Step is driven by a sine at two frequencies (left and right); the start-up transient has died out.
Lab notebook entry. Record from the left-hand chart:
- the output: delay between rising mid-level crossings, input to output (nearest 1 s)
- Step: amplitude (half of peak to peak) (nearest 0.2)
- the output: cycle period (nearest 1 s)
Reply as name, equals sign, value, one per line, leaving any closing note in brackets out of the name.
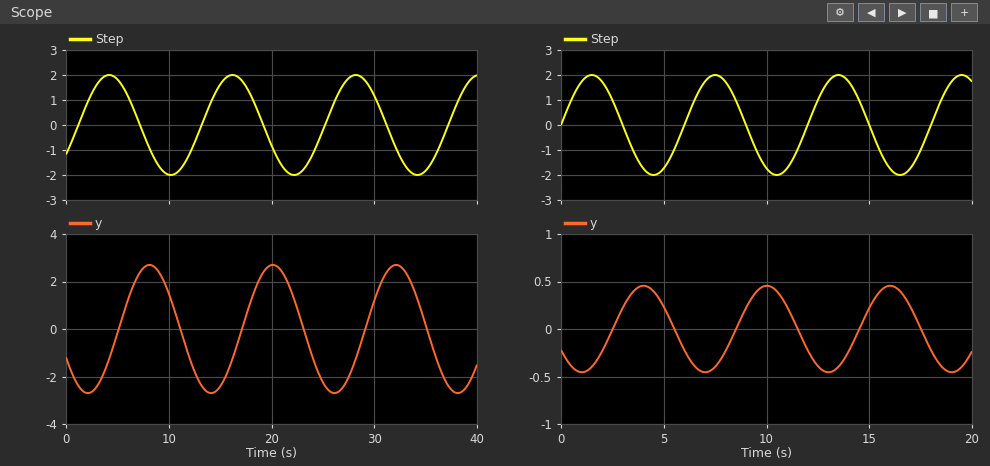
the output: delay between rising mid-level crossings, input to output = 4 s
Step: amplitude (half of peak to peak) = 2.0
the output: cycle period = 12 s
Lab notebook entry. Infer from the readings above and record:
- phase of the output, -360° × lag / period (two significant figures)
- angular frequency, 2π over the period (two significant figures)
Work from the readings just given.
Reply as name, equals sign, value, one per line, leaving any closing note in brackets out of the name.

phase of the output, -360° × lag / period = -120°
angular frequency, 2π over the period = 0.52 rad/s
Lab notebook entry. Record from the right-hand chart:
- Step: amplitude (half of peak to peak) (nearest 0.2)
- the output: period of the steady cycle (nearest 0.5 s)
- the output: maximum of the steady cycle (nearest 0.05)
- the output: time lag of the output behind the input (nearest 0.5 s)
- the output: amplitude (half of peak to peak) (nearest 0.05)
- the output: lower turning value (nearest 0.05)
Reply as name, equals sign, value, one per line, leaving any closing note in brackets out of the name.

Step: amplitude (half of peak to peak) = 2.0
the output: period of the steady cycle = 6.0 s
the output: maximum of the steady cycle = 0.45
the output: time lag of the output behind the input = 2.5 s
the output: amplitude (half of peak to peak) = 0.45
the output: lower turning value = -0.45
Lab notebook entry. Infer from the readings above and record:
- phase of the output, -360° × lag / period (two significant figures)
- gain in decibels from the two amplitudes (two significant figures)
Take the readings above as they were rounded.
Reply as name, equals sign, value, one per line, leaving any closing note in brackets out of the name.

phase of the output, -360° × lag / period = -150°
gain in decibels from the two amplitudes = -13 dB
